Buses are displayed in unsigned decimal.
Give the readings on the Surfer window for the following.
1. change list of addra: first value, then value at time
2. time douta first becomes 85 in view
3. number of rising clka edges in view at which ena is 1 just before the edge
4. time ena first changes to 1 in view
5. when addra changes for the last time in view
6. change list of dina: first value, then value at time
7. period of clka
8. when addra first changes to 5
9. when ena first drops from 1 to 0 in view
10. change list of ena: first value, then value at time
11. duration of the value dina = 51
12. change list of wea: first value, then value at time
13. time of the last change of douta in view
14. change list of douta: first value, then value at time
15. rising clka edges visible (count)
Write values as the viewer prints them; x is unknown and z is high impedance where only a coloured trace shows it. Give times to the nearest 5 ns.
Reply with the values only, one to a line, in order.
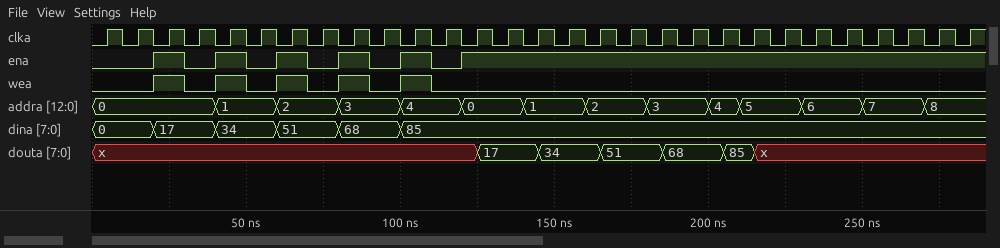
0, 1 at 40 ns, 2 at 60 ns, 3 at 80 ns, 4 at 100 ns, 0 at 120 ns, 1 at 140 ns, 2 at 160 ns, 3 at 180 ns, 4 at 200 ns, 5 at 210 ns, 6 at 230 ns, 7 at 250 ns, 8 at 270 ns
205 ns
22
20 ns
270 ns
0, 17 at 20 ns, 34 at 40 ns, 51 at 60 ns, 68 at 80 ns, 85 at 100 ns
10 ns
210 ns
30 ns
0, 1 at 20 ns, 0 at 30 ns, 1 at 40 ns, 0 at 50 ns, 1 at 60 ns, 0 at 70 ns, 1 at 80 ns, 0 at 90 ns, 1 at 100 ns, 0 at 110 ns, 1 at 120 ns
20 ns
0, 1 at 20 ns, 0 at 30 ns, 1 at 40 ns, 0 at 50 ns, 1 at 60 ns, 0 at 70 ns, 1 at 80 ns, 0 at 90 ns, 1 at 100 ns, 0 at 110 ns
215 ns
x, 17 at 125 ns, 34 at 145 ns, 51 at 165 ns, 68 at 185 ns, 85 at 205 ns, x at 215 ns
29
